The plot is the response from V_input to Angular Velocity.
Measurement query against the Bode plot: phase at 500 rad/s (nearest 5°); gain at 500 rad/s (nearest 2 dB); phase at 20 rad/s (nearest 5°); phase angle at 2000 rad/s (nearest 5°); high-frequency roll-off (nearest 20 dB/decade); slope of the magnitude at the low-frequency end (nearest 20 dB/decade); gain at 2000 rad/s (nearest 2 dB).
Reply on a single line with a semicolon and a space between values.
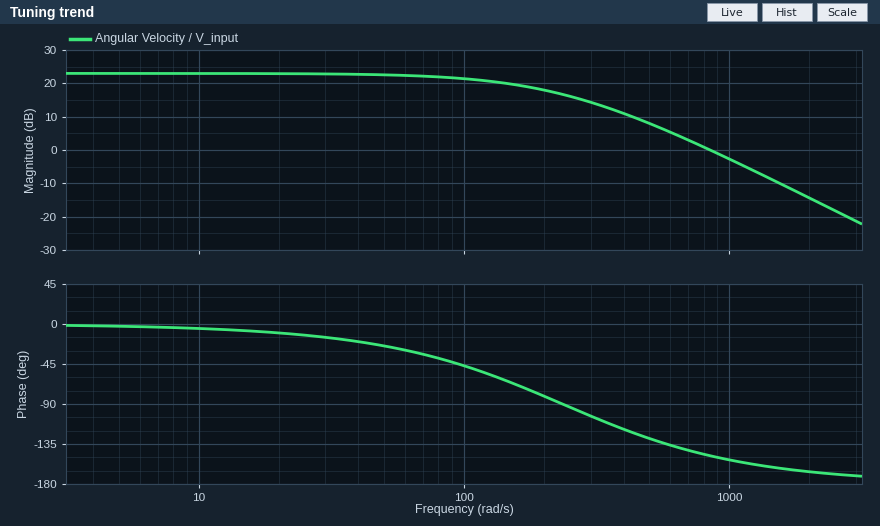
-130°; 8 dB; -10°; -165°; -40 dB/decade; 0 dB/decade; -14 dB
